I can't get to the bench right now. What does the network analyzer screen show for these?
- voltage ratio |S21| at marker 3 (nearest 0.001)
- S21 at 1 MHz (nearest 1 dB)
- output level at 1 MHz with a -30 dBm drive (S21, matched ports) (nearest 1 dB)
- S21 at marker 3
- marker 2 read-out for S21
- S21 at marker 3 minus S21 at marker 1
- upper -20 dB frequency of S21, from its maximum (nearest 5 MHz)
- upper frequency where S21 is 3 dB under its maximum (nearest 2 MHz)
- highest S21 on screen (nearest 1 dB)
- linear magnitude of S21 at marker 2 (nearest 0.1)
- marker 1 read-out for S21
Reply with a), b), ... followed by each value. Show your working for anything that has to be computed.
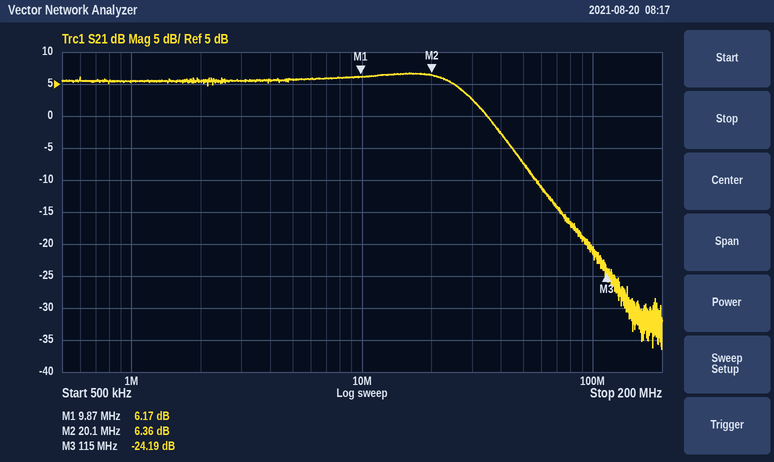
a) 10^(-24.19/20) ≈ 0.062
b) 5 dB
c) -30 dBm + (5 dB) = -25 dBm
d) -24.19 dB
e) 6.36 dB
f) -24.19 − (6.17) = -30.36 dB
g) 65 MHz
h) 28 MHz
i) 7 dB
j) 10^(6.36/20) ≈ 2.1
k) 6.17 dB
